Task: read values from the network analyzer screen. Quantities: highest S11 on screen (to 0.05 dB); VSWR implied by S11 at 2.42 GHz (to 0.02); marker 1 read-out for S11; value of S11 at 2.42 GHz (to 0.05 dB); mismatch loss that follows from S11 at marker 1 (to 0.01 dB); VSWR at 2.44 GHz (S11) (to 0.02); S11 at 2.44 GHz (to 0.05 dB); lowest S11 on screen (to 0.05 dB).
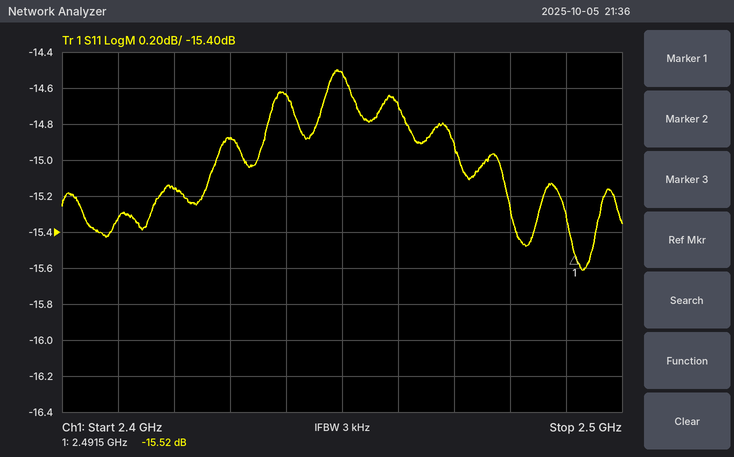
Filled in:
-14.50 dB
1.42
-15.52 dB
-15.15 dB
0.12 dB
1.46
-14.65 dB
-15.60 dB
